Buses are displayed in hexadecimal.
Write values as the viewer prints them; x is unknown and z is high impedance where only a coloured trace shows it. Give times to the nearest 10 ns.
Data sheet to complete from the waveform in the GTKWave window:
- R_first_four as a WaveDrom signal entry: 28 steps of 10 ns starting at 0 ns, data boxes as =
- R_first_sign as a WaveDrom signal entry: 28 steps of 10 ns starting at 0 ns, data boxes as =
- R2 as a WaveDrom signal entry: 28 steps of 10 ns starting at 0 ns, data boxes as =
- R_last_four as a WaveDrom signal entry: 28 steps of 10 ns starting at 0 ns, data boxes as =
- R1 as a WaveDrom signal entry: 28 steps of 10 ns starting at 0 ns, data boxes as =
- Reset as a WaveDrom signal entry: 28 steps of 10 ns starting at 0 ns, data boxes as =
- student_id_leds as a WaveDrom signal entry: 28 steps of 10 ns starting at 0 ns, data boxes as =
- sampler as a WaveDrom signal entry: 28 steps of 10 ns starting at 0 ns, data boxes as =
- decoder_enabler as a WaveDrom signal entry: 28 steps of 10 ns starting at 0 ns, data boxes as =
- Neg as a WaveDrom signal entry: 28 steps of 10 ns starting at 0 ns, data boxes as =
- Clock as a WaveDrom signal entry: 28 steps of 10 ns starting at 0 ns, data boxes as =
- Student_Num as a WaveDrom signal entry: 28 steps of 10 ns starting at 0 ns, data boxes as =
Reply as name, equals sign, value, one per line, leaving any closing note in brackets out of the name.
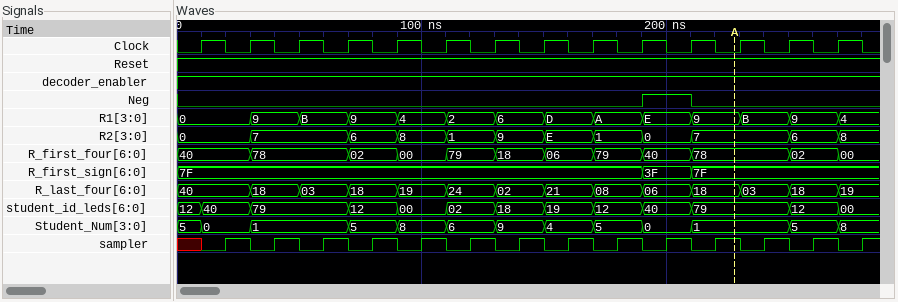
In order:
R_first_four as a WaveDrom signal entry: 28 steps of 10 ns starting at 0 ns, data boxes as = = {name: 'R_first_four', wave: '=..=...=.=.=.=.=.=.=.=...=.=', data: '40 78 02 00 79 18 06 79 40 78 02 00'}
R_first_sign as a WaveDrom signal entry: 28 steps of 10 ns starting at 0 ns, data boxes as = = {name: 'R_first_sign', wave: '=..................=.=......', data: '7F 3F 7F'}
R2 as a WaveDrom signal entry: 28 steps of 10 ns starting at 0 ns, data boxes as = = {name: 'R2', wave: '=..=...=.=.=.=.=.=.=.=...=.=', data: '0 7 6 8 1 9 E 1 0 7 6 8'}
R_last_four as a WaveDrom signal entry: 28 steps of 10 ns starting at 0 ns, data boxes as = = {name: 'R_last_four', wave: '=..=.=.=.=.=.=.=.=.=.=.=.=.=', data: '40 18 03 18 19 24 02 21 08 06 18 03 18 19'}
R1 as a WaveDrom signal entry: 28 steps of 10 ns starting at 0 ns, data boxes as = = {name: 'R1', wave: '=..=.=.=.=.=.=.=.=.=.=.=.=.=', data: '0 9 B 9 4 2 6 D A E 9 B 9 4'}
Reset as a WaveDrom signal entry: 28 steps of 10 ns starting at 0 ns, data boxes as = = {name: 'Reset', wave: '1...........................'}
student_id_leds as a WaveDrom signal entry: 28 steps of 10 ns starting at 0 ns, data boxes as = = {name: 'student_id_leds', wave: '==.=...=.=.=.=.=.=.=.=...=.=', data: '12 40 79 12 00 02 18 19 12 40 79 12 00'}
sampler as a WaveDrom signal entry: 28 steps of 10 ns starting at 0 ns, data boxes as = = {name: 'sampler', wave: 'x010101010101010101010101010'}
decoder_enabler as a WaveDrom signal entry: 28 steps of 10 ns starting at 0 ns, data boxes as = = {name: 'decoder_enabler', wave: '1...........................'}
Neg as a WaveDrom signal entry: 28 steps of 10 ns starting at 0 ns, data boxes as = = {name: 'Neg', wave: '0..................1.0......'}
Clock as a WaveDrom signal entry: 28 steps of 10 ns starting at 0 ns, data boxes as = = {name: 'Clock', wave: '0101010101010101010101010101'}
Student_Num as a WaveDrom signal entry: 28 steps of 10 ns starting at 0 ns, data boxes as = = {name: 'Student_Num', wave: '==.=...=.=.=.=.=.=.=.=...=.=', data: '5 0 1 5 8 6 9 4 5 0 1 5 8'}
